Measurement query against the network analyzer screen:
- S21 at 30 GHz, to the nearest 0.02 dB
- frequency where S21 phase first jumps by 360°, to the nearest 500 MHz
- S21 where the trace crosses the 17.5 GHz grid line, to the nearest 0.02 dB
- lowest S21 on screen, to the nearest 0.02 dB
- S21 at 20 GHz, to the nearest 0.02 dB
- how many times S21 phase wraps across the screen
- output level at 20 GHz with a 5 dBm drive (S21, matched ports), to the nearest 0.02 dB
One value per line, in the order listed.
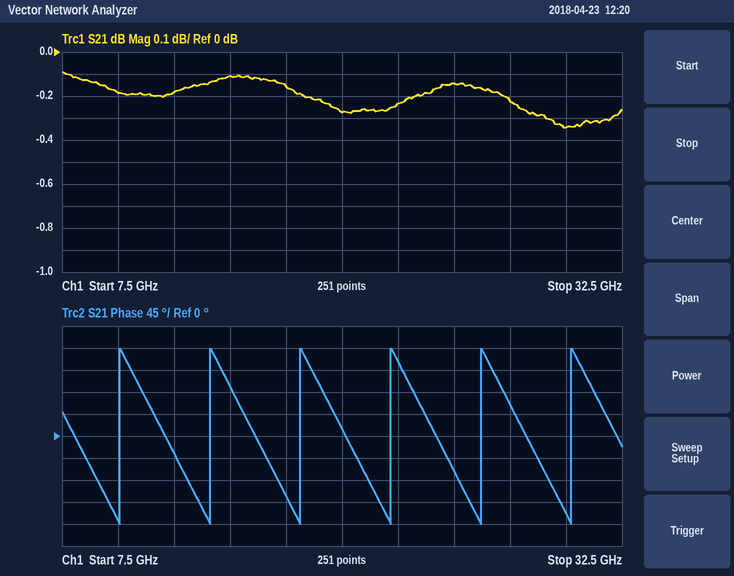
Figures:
-0.34 dB
10.0 GHz
-0.16 dB
-0.34 dB
-0.28 dB
6
4.72 dBm
